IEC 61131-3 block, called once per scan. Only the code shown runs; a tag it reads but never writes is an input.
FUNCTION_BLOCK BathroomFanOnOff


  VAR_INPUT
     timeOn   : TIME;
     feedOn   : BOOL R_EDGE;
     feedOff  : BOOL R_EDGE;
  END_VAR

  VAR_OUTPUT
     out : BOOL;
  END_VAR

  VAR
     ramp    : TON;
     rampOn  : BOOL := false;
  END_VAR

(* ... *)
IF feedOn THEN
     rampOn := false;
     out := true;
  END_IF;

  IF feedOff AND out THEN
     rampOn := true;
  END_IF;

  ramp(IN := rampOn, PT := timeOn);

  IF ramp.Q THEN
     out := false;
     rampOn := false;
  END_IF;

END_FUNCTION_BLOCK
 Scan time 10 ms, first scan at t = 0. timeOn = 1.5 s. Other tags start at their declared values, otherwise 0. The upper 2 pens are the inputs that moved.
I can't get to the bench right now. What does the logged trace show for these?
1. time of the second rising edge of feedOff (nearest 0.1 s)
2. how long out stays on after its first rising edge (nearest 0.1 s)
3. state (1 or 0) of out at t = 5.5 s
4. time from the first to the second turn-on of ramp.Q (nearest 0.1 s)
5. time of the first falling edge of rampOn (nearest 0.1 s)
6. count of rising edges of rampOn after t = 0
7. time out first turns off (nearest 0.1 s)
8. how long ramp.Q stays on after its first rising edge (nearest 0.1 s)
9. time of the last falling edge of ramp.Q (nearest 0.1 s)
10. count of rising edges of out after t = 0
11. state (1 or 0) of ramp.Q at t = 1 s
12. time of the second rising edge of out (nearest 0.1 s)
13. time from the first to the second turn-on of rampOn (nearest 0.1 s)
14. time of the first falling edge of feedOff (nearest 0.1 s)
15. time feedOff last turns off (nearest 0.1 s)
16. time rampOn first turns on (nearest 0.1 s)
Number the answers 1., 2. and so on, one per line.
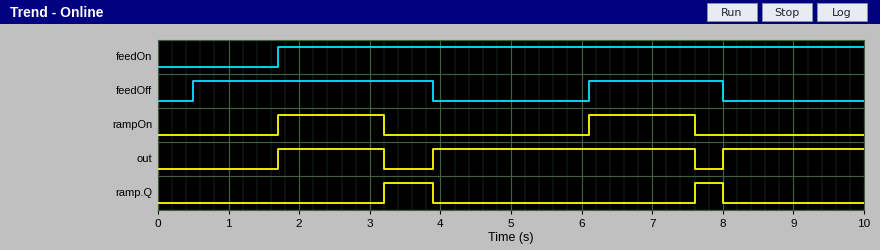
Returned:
1. 6.1 s
2. 1.5 s
3. 1
4. 4.4 s
5. 3.2 s
6. 2
7. 3.2 s
8. 0.7 s
9. 8.0 s
10. 3
11. 0
12. 3.9 s
13. 4.4 s
14. 3.9 s
15. 8.0 s
16. 1.7 s
